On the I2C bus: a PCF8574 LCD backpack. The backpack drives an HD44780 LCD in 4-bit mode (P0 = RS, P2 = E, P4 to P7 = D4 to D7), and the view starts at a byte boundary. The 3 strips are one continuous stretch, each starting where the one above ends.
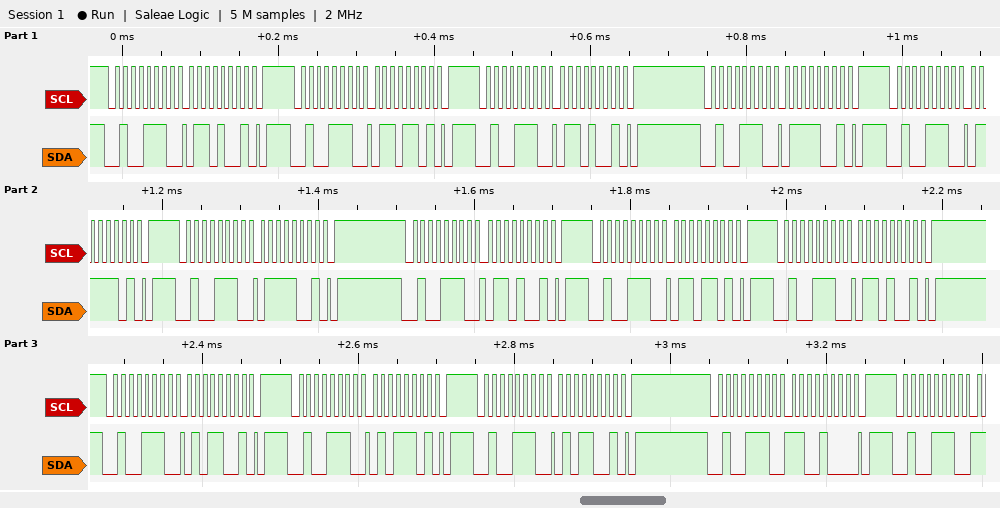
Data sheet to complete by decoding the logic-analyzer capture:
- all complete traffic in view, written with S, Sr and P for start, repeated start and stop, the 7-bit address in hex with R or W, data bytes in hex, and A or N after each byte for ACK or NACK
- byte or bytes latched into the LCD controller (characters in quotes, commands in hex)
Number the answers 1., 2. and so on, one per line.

1. S 27W A 69 A P S 27W A 6D A P S 27W A 69 A P S 27W A 79 A P S 27W A 7D A P S 27W A 79 A P S 27W A 69 A P S 27W A 6D A P S 27W A 69 A P S 27W A 59 A P S 27W A 5D A P S 27W A 59 A P S 27W A C8 A P S 27W A
2. 'g' 'e'
